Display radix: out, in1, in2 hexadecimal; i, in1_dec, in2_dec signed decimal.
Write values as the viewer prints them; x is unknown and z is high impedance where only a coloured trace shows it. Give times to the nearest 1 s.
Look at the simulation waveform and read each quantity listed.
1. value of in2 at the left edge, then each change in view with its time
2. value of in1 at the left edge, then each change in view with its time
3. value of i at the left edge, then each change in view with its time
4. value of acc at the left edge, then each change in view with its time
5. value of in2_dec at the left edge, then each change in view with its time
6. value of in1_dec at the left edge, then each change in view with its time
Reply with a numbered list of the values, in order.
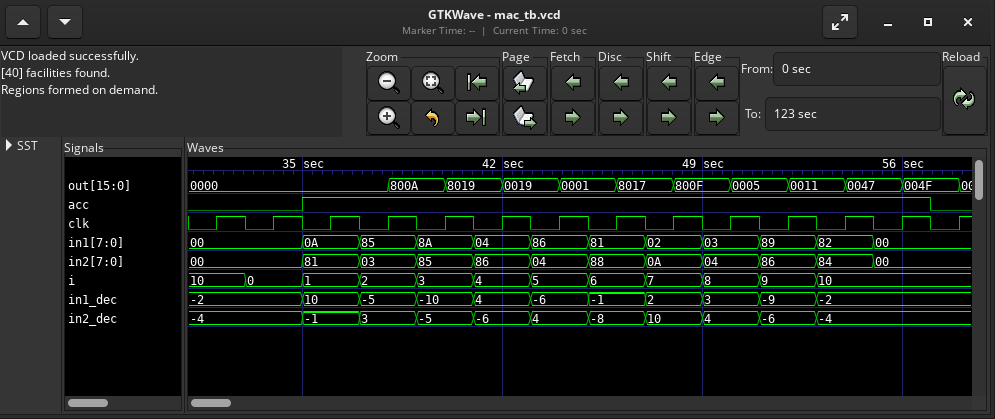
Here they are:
1. 00, 81 at 35 s, 03 at 37 s, 85 at 39 s, 86 at 41 s, 04 at 43 s, 88 at 45 s, 0A at 47 s, 04 at 49 s, 86 at 51 s, 84 at 53 s, 00 at 55 s
2. 00, 0A at 35 s, 85 at 37 s, 8A at 39 s, 04 at 41 s, 86 at 43 s, 81 at 45 s, 02 at 47 s, 03 at 49 s, 89 at 51 s, 82 at 53 s, 00 at 55 s
3. 10, 0 at 33 s, 1 at 35 s, 2 at 37 s, 3 at 39 s, 4 at 41 s, 5 at 43 s, 6 at 45 s, 7 at 47 s, 8 at 49 s, 9 at 51 s, 10 at 53 s
4. 0, 1 at 35 s, 0 at 57 s
5. -4, -1 at 35 s, 3 at 37 s, -5 at 39 s, -6 at 41 s, 4 at 43 s, -8 at 45 s, 10 at 47 s, 4 at 49 s, -6 at 51 s, -4 at 53 s
6. -2, 10 at 35 s, -5 at 37 s, -10 at 39 s, 4 at 41 s, -6 at 43 s, -1 at 45 s, 2 at 47 s, 3 at 49 s, -9 at 51 s, -2 at 53 s
